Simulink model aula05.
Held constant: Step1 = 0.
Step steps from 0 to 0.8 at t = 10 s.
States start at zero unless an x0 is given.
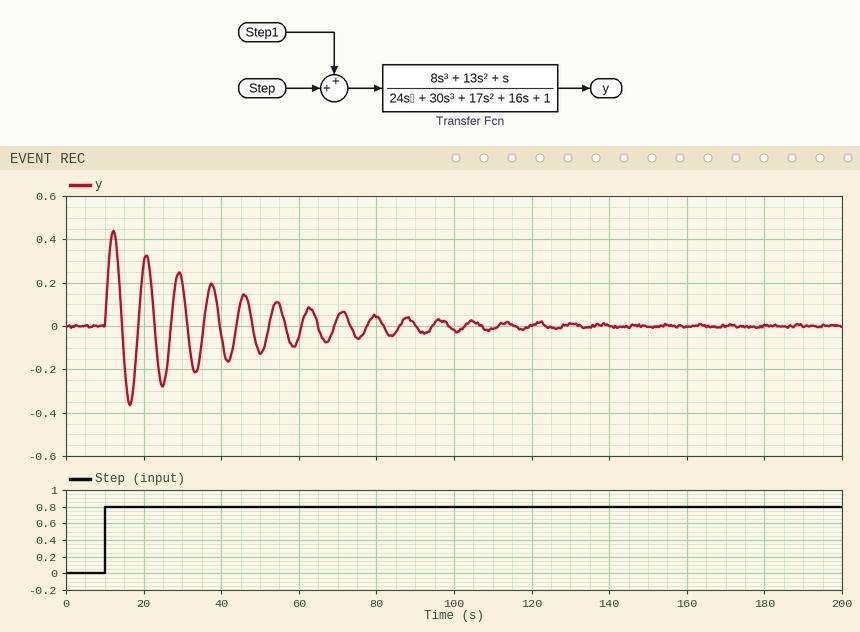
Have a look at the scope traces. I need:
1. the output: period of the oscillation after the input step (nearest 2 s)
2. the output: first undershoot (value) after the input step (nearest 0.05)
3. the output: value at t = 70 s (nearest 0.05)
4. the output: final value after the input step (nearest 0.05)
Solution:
8 s
-0.35
0.05
0.00
